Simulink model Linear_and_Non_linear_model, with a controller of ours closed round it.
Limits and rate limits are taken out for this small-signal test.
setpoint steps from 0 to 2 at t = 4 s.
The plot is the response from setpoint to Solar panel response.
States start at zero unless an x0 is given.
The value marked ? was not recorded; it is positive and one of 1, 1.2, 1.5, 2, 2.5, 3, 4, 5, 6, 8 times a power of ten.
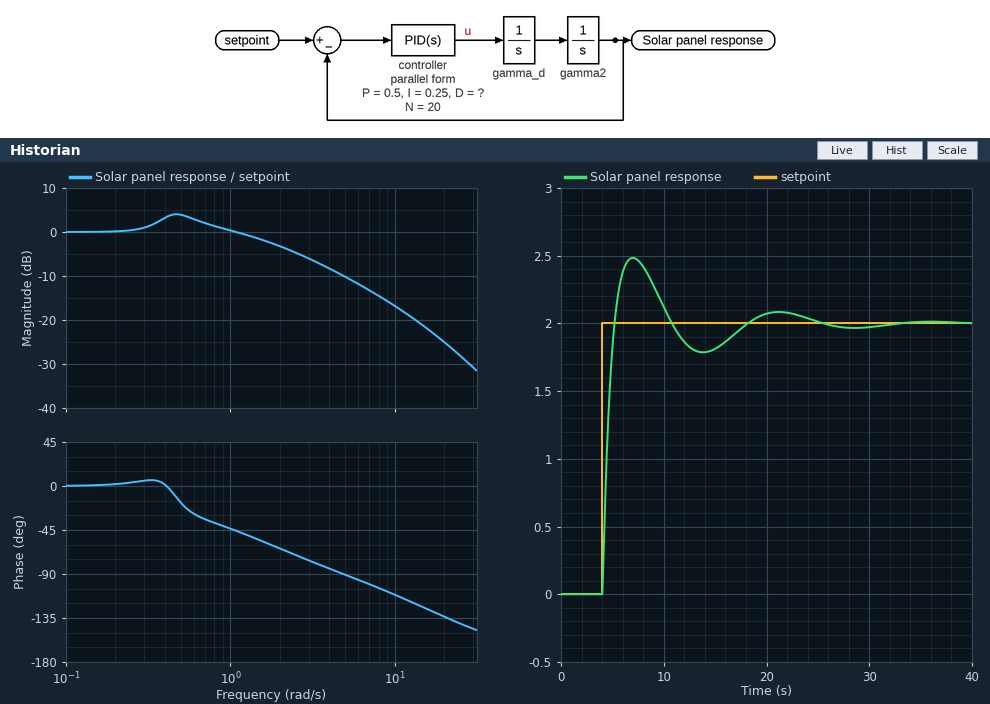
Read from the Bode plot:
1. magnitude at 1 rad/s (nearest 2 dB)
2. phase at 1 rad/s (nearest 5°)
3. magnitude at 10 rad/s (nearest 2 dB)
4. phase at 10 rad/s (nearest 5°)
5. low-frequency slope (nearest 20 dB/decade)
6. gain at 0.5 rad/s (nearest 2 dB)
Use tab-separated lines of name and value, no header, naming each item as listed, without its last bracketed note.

magnitude at 1 rad/s	0 dB
phase at 1 rad/s	-45°
magnitude at 10 rad/s	-16 dB
phase at 10 rad/s	-110°
low-frequency slope	0 dB/decade
gain at 0.5 rad/s	4 dB
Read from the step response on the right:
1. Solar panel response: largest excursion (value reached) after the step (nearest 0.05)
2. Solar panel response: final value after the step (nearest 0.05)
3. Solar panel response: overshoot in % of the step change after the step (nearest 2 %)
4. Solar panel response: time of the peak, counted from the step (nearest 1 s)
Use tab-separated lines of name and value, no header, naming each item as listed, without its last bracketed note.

Solar panel response: largest excursion (value reached) after the step	2.50
Solar panel response: final value after the step	2.00
Solar panel response: overshoot in % of the step change after the step	24 %
Solar panel response: time of the peak, counted from the step	3 s
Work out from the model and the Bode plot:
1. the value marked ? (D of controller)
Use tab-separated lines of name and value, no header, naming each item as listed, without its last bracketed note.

the value marked ?	1.5
